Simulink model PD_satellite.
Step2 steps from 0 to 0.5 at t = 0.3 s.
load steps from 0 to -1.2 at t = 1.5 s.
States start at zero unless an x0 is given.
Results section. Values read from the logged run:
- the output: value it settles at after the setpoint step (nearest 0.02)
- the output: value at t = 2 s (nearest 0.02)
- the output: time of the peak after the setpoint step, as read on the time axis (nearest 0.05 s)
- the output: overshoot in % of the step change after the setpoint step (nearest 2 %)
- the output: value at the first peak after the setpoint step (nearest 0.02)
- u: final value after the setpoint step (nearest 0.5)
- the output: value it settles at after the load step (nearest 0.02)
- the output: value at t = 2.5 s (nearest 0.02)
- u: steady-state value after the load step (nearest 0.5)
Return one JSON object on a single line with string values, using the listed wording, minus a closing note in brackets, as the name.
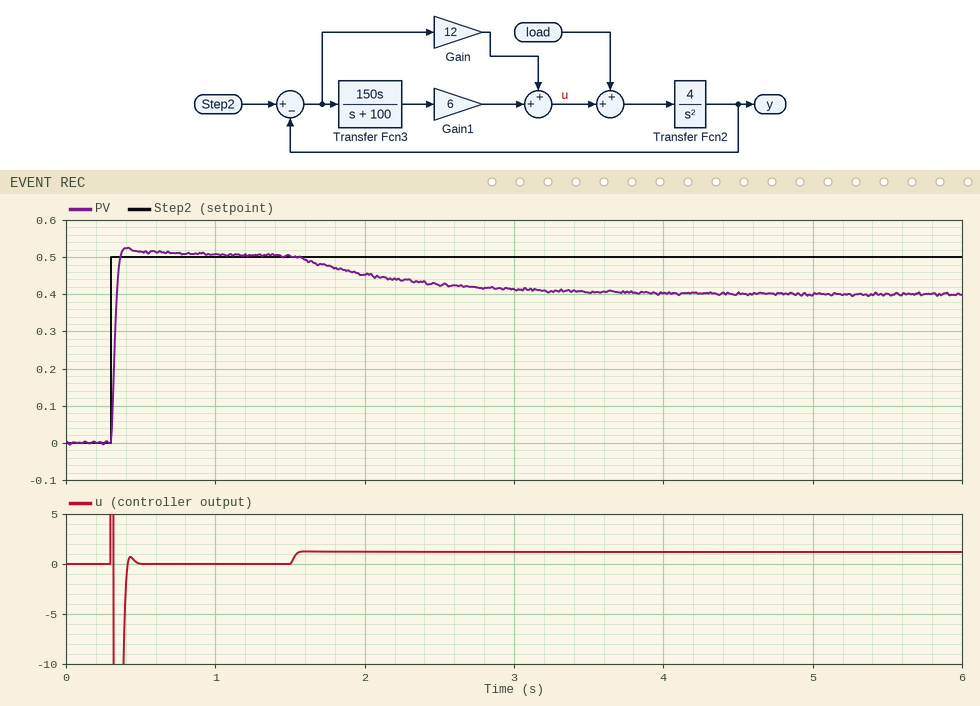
{"the output: value it settles at after the setpoint step": "0.50", "the output: value at t = 2 s": "0.46", "the output: time of the peak after the setpoint step, as read on the time axis": "0.40 s", "the output: overshoot in % of the step change after the setpoint step": "4 %", "the output: value at the first peak after the setpoint step": "0.52", "u: final value after the setpoint step": "0.0", "the output: value it settles at after the load step": "0.40", "the output: value at t = 2.5 s": "0.42", "u: steady-state value after the load step": "1.0"}
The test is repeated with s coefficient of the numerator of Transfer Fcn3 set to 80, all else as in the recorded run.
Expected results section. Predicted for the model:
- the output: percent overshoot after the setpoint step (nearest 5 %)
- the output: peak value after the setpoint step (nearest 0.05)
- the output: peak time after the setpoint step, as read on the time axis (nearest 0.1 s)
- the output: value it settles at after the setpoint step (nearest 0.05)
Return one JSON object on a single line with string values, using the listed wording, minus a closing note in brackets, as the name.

{"the output: percent overshoot after the setpoint step": "10 %", "the output: peak value after the setpoint step": "0.55", "the output: peak time after the setpoint step, as read on the time axis": "0.5 s", "the output: value it settles at after the setpoint step": "0.50"}
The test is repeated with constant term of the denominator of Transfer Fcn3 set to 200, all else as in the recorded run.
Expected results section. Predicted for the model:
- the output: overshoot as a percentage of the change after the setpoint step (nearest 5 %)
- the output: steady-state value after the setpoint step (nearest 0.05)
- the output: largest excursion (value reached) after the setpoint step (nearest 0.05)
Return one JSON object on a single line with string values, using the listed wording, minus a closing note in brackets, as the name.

{"the output: overshoot as a percentage of the change after the setpoint step": "10 %", "the output: steady-state value after the setpoint step": "0.50", "the output: largest excursion (value reached) after the setpoint step": "0.55"}
